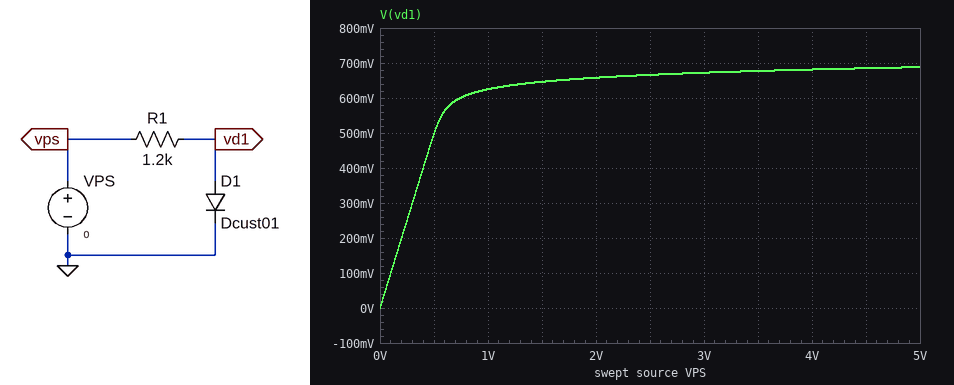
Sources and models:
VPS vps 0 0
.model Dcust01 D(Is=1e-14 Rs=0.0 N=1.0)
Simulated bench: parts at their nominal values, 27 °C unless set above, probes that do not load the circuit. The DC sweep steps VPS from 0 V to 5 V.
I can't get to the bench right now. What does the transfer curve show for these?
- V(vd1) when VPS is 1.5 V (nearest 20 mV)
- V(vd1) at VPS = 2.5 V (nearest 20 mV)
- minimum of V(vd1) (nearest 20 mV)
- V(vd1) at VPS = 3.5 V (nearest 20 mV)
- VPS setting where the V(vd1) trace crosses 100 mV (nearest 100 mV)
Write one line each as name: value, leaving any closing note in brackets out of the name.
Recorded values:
V(vd1) when VPS is 1.5 V: 640 mV
V(vd1) at VPS = 2.5 V: 660 mV
minimum of V(vd1): 0 V
V(vd1) at VPS = 3.5 V: 680 mV
VPS setting where the V(vd1) trace crosses 100 mV: 100 mV
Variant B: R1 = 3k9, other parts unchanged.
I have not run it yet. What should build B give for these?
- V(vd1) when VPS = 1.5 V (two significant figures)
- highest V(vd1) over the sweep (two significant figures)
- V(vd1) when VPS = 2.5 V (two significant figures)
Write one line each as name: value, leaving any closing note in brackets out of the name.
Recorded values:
V(vd1) when VPS = 1.5 V: 620 mV
highest V(vd1) over the sweep: 660 mV
V(vd1) when VPS = 2.5 V: 640 mV
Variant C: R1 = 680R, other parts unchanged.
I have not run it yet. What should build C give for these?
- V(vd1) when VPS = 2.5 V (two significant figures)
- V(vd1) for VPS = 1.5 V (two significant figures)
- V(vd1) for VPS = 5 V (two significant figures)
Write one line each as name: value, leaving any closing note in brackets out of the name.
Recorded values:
V(vd1) when VPS = 2.5 V: 680 mV
V(vd1) for VPS = 1.5 V: 660 mV
V(vd1) for VPS = 5 V: 700 mV
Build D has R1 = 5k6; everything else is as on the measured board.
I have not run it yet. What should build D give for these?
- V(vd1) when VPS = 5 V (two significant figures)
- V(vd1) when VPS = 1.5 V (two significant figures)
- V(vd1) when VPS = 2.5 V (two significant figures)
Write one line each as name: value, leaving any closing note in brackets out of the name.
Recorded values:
V(vd1) when VPS = 5 V: 650 mV
V(vd1) when VPS = 1.5 V: 610 mV
V(vd1) when VPS = 2.5 V: 630 mV
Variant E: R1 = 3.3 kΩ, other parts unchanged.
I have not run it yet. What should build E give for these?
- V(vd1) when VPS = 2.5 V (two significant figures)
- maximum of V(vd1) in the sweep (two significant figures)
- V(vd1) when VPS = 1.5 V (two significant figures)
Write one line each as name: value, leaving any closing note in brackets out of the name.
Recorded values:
V(vd1) when VPS = 2.5 V: 640 mV
maximum of V(vd1) in the sweep: 660 mV
V(vd1) when VPS = 1.5 V: 620 mV
